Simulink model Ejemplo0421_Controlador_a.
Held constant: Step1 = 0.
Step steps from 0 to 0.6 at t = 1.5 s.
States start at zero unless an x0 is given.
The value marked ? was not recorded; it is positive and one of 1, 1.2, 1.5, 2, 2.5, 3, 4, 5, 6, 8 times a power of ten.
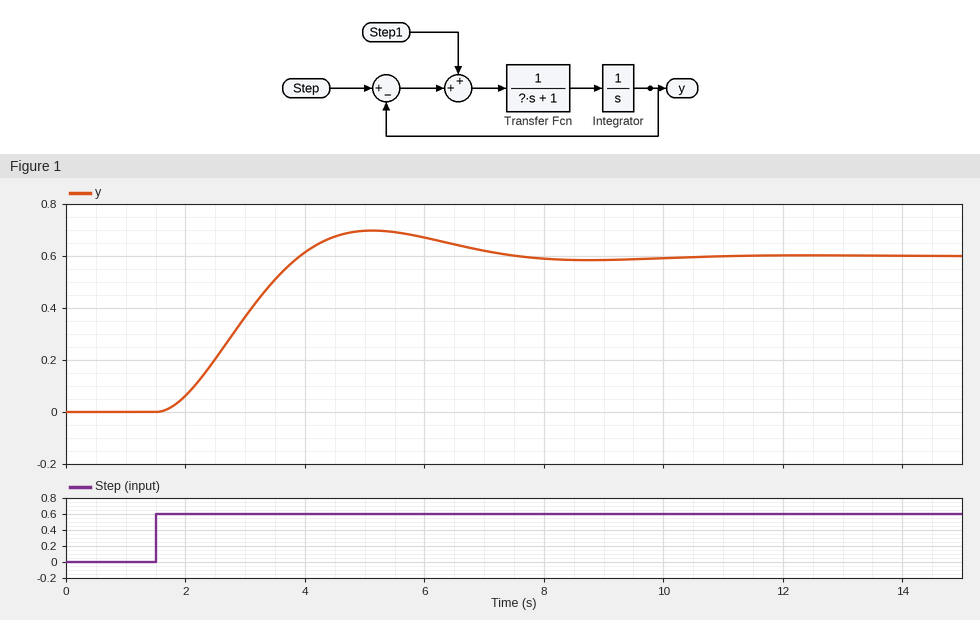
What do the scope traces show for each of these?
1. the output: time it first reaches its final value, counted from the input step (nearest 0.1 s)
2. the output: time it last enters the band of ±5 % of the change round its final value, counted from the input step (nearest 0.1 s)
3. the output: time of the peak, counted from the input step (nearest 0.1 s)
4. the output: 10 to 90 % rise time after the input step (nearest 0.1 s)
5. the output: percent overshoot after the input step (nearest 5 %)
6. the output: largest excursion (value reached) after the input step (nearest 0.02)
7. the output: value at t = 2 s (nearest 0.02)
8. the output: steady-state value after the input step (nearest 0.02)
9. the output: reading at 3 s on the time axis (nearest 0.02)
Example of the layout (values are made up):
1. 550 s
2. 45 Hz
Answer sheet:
1. 2.4 s
2. 5.3 s
3. 3.6 s
4. 1.6 s
5. 15 %
6. 0.70
7. 0.06
8. 0.60
9. 0.36
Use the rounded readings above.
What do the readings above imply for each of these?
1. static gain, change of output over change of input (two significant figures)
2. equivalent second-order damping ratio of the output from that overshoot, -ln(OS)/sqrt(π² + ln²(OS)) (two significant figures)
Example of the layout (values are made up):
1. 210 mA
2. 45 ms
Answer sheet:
1. 1.0
2. 0.52
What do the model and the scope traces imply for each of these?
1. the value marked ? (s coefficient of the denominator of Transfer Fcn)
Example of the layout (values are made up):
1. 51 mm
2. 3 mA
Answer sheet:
1. 1
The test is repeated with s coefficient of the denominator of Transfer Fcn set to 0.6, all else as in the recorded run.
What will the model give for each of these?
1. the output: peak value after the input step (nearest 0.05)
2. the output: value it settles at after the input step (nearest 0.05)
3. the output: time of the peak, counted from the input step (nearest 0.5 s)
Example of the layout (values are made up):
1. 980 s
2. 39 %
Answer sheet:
1. 0.65
2. 0.60
3. 3.0 s
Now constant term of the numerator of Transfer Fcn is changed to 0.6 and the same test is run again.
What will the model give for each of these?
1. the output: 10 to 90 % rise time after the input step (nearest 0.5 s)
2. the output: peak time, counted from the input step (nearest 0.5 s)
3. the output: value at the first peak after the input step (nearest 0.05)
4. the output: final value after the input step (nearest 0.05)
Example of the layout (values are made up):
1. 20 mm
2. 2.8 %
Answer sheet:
1. 2.5 s
2. 5.5 s
3. 0.65
4. 0.60
